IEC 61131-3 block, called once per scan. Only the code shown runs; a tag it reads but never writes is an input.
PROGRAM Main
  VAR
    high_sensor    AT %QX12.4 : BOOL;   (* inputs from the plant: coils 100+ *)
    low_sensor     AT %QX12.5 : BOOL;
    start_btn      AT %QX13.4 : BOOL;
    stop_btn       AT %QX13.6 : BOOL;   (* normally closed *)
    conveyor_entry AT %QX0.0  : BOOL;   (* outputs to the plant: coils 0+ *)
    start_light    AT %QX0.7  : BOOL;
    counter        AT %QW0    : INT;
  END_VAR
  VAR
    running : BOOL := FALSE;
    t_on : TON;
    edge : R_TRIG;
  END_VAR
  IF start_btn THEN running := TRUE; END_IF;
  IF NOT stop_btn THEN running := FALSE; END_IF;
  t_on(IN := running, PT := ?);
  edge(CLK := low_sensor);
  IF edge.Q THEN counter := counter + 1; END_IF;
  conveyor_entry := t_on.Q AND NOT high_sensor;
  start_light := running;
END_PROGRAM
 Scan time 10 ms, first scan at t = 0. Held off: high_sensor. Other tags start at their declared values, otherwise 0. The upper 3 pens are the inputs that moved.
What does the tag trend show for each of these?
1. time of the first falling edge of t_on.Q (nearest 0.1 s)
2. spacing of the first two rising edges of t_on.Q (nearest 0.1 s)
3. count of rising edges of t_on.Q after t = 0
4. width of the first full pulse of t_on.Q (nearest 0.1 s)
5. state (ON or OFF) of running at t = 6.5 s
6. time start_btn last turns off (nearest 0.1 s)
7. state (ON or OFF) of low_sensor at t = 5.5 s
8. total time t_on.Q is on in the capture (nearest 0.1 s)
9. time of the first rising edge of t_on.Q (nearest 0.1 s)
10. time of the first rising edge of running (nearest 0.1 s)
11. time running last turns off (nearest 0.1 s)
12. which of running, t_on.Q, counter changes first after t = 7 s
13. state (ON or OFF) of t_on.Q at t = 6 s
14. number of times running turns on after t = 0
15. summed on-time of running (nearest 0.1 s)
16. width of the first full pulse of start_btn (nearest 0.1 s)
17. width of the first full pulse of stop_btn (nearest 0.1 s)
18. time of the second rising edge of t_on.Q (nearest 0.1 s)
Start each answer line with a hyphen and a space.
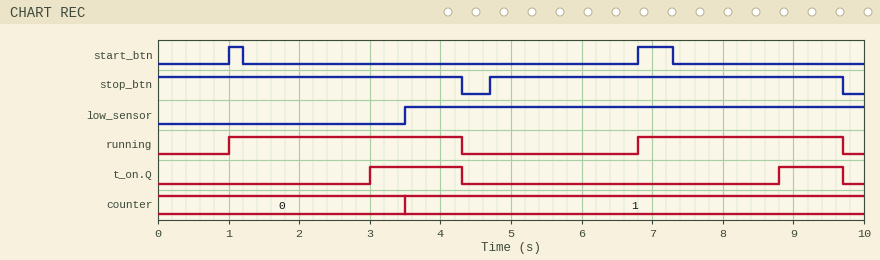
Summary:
- 4.3 s
- 5.8 s
- 2
- 1.3 s
- OFF
- 7.3 s
- ON
- 2.2 s
- 3.0 s
- 1.0 s
- 9.7 s
- t_on.Q
- OFF
- 2
- 6.2 s
- 0.2 s
- 5.0 s
- 8.8 s
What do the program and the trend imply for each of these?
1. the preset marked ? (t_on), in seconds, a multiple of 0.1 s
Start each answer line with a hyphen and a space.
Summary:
- 2.0 s
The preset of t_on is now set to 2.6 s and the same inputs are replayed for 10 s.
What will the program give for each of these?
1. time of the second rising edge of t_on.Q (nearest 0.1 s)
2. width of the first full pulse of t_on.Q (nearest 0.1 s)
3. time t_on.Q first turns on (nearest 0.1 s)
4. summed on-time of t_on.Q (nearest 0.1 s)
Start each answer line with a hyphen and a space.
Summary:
- 9.4 s
- 0.7 s
- 3.6 s
- 1.0 s
